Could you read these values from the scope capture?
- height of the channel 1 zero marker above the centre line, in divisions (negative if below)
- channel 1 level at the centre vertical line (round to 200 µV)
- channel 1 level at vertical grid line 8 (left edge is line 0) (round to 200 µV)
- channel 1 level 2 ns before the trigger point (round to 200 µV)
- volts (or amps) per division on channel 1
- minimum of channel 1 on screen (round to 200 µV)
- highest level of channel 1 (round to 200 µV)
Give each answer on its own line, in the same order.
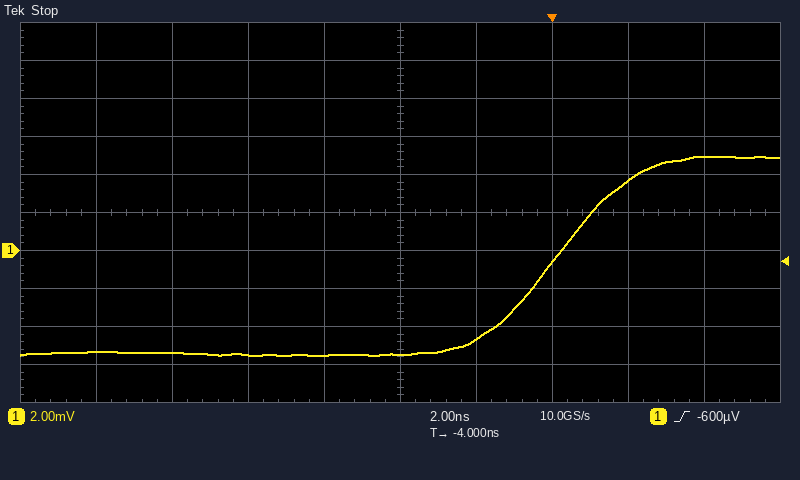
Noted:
-1.0 div
-5.4 mV
3.6 mV
-4.6 mV
2 mV
-5.6 mV
5.0 mV
